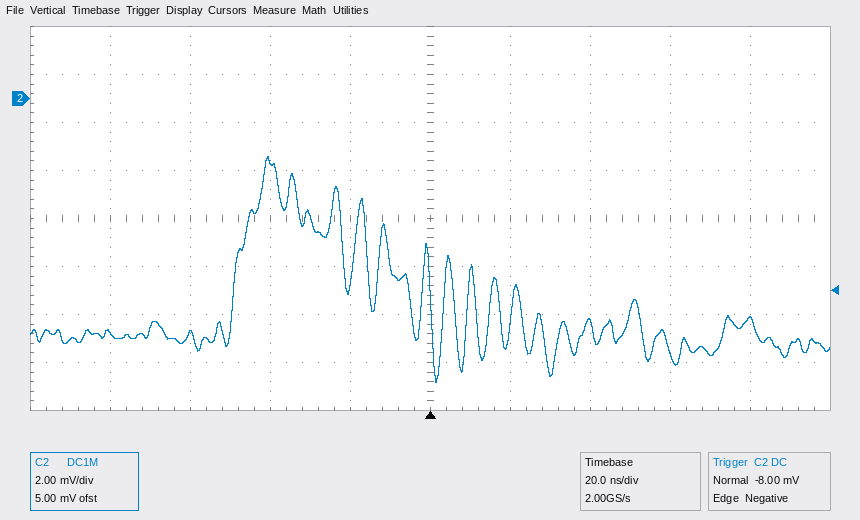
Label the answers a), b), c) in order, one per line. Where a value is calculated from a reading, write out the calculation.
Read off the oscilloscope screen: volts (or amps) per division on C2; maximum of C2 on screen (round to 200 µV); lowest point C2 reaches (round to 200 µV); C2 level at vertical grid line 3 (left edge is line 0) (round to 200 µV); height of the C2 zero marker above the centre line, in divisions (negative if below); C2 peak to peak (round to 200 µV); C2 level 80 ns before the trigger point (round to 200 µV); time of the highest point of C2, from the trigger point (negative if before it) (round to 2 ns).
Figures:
a) 2 mV
b) -2.4 mV
c) -11.8 mV
d) -2.6 mV
e) +2.5 div
f) -2.4 mV − (-11.8 mV) = 9.4 mV
g) -9.8 mV
h) -40 ns
